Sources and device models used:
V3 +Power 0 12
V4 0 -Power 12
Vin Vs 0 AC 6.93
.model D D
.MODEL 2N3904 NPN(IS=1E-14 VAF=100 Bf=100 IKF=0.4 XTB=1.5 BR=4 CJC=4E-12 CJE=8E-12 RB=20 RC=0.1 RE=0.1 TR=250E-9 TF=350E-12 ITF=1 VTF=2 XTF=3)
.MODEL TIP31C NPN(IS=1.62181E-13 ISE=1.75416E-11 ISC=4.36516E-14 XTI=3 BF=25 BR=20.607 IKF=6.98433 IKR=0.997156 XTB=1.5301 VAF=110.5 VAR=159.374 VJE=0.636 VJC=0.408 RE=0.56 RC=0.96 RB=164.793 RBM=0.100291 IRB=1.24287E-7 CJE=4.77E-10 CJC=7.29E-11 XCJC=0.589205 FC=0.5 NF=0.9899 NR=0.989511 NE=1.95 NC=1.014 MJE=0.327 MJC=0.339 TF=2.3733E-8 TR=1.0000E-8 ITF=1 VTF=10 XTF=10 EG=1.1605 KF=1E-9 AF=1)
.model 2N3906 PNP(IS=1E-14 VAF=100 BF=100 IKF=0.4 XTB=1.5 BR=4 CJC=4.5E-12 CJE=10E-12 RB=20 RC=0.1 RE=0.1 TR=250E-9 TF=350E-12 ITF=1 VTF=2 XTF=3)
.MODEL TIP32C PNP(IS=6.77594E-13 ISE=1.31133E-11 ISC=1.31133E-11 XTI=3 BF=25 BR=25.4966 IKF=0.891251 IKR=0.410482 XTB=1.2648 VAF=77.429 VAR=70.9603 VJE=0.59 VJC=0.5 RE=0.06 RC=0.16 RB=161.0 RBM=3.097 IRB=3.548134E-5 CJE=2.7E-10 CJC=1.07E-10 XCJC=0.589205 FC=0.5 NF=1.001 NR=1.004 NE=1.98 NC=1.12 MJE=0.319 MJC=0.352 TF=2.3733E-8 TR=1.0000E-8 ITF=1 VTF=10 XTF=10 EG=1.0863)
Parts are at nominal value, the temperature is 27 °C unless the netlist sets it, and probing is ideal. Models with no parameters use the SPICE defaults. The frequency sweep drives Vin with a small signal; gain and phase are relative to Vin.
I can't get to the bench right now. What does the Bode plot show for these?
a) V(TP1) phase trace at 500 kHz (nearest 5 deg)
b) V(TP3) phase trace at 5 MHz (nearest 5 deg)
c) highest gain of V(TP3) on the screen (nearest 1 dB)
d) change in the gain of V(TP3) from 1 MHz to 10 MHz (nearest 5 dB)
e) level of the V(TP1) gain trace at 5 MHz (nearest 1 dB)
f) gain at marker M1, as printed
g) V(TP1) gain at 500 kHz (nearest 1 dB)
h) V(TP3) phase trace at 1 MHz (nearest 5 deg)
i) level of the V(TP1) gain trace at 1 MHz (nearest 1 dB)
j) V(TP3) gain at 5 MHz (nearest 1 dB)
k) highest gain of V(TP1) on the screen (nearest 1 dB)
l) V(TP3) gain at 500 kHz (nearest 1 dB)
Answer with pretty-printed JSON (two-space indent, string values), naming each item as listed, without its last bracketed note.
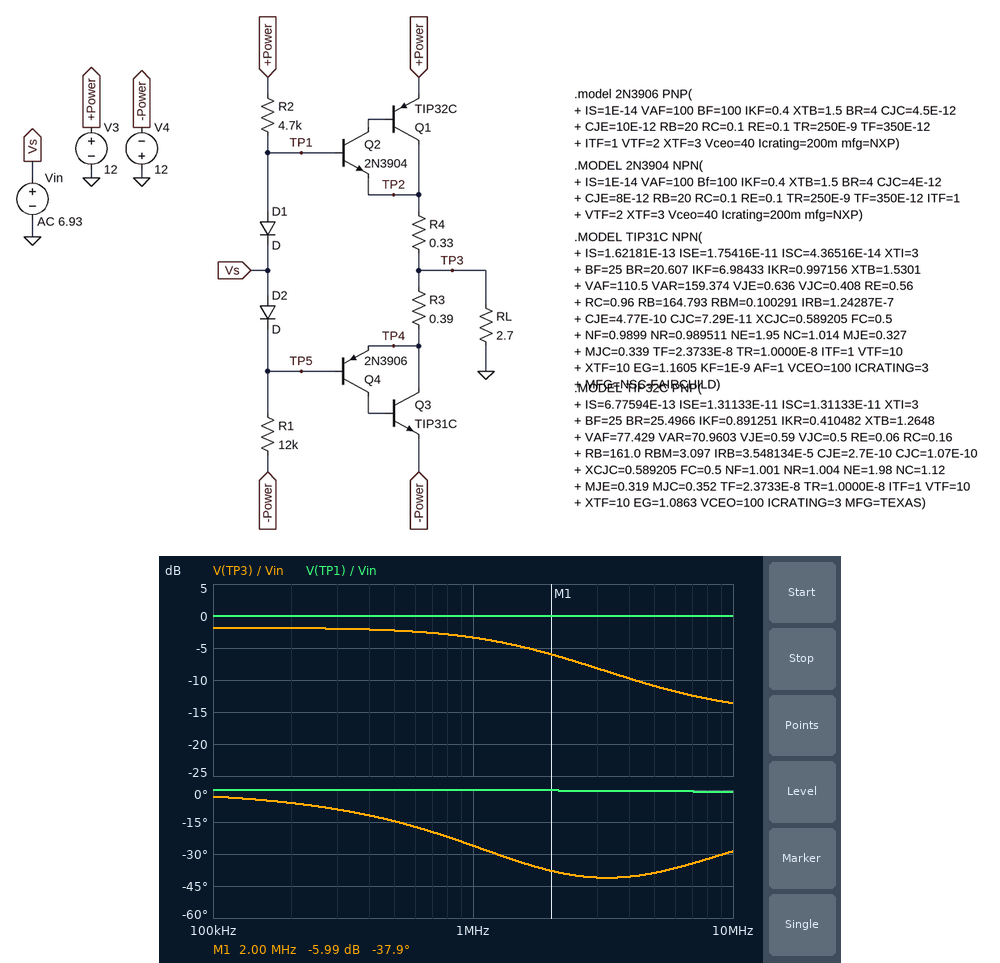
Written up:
{
  "V(TP1) phase trace at 500 kHz": "0 deg",
  "V(TP3) phase trace at 5 MHz": "-40 deg",
  "highest gain of V(TP3) on the screen": "-2 dB",
  "change in the gain of V(TP3) from 1 MHz to 10 MHz": "-10 dB",
  "level of the V(TP1) gain trace at 5 MHz": "0 dB",
  "gain at marker M1, as printed": "-5.99 dB",
  "V(TP1) gain at 500 kHz": "0 dB",
  "V(TP3) phase trace at 1 MHz": "-25 deg",
  "level of the V(TP1) gain trace at 1 MHz": "0 dB",
  "V(TP3) gain at 5 MHz": "-11 dB",
  "highest gain of V(TP1) on the screen": "0 dB",
  "V(TP3) gain at 500 kHz": "-2 dB"
}
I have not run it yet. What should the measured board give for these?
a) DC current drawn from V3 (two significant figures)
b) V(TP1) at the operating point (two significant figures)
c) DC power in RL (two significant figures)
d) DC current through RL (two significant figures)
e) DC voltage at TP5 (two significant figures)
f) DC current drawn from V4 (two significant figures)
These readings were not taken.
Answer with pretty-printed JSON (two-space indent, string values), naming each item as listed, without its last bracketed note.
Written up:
{
  "DC current drawn from V3": "35 mA",
  "V(TP1) at the operating point": "680 mV",
  "DC power in RL": "43 µW",
  "DC current through RL": "4.0 mA",
  "DC voltage at TP5": "-650 mV",
  "DC current drawn from V4": "29 mA"
}
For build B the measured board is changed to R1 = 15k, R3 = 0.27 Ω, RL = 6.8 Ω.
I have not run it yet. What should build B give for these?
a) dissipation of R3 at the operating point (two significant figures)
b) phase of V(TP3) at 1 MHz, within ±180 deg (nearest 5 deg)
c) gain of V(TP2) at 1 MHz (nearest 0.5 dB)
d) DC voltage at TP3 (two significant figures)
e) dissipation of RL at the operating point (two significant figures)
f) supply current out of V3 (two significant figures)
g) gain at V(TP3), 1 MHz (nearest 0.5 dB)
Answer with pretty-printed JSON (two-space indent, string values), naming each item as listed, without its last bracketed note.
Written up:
{
  "dissipation of R3 at the operating point": "220 µW",
  "phase of V(TP3) at 1 MHz, within ±180 deg": "-15 deg",
  "gain of V(TP2) at 1 MHz": "-1.0 dB",
  "DC voltage at TP3": "13 mV",
  "dissipation of RL at the operating point": "26 µW",
  "supply current out of V3": "33 mA",
  "gain at V(TP3), 1 MHz": "-1.5 dB"
}
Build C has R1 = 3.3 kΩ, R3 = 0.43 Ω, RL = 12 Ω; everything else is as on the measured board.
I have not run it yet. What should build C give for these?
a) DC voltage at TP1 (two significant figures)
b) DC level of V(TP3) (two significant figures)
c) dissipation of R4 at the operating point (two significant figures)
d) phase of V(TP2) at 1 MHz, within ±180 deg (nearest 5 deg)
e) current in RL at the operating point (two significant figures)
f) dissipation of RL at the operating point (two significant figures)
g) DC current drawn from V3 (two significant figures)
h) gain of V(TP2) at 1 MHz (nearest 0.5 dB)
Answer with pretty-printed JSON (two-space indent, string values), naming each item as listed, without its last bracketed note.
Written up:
{
  "DC voltage at TP1": "680 mV",
  "DC level of V(TP3)": "-2.2 mV",
  "dissipation of R4 at the operating point": "670 µW",
  "phase of V(TP2) at 1 MHz, within ±180 deg": "-5 deg",
  "current in RL at the operating point": "180 µA",
  "dissipation of RL at the operating point": "400 nW",
  "DC current drawn from V3": "47 mA",
  "gain of V(TP2) at 1 MHz": "-0.5 dB"
}
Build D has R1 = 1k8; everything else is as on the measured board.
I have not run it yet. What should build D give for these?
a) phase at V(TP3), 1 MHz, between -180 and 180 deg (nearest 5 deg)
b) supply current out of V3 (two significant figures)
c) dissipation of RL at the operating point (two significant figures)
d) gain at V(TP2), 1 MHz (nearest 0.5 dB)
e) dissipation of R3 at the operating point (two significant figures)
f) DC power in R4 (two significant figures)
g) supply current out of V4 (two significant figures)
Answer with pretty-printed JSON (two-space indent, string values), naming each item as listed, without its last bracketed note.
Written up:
{
  "phase at V(TP3), 1 MHz, between -180 and 180 deg": "-15 deg",
  "supply current out of V3": "55 mA",
  "dissipation of RL at the operating point": "32 µW",
  "gain at V(TP2), 1 MHz": "-1.5 dB",
  "dissipation of R3 at the operating point": "1.2 mW",
  "DC power in R4": "920 µW",
  "supply current out of V4": "63 mA"
}
